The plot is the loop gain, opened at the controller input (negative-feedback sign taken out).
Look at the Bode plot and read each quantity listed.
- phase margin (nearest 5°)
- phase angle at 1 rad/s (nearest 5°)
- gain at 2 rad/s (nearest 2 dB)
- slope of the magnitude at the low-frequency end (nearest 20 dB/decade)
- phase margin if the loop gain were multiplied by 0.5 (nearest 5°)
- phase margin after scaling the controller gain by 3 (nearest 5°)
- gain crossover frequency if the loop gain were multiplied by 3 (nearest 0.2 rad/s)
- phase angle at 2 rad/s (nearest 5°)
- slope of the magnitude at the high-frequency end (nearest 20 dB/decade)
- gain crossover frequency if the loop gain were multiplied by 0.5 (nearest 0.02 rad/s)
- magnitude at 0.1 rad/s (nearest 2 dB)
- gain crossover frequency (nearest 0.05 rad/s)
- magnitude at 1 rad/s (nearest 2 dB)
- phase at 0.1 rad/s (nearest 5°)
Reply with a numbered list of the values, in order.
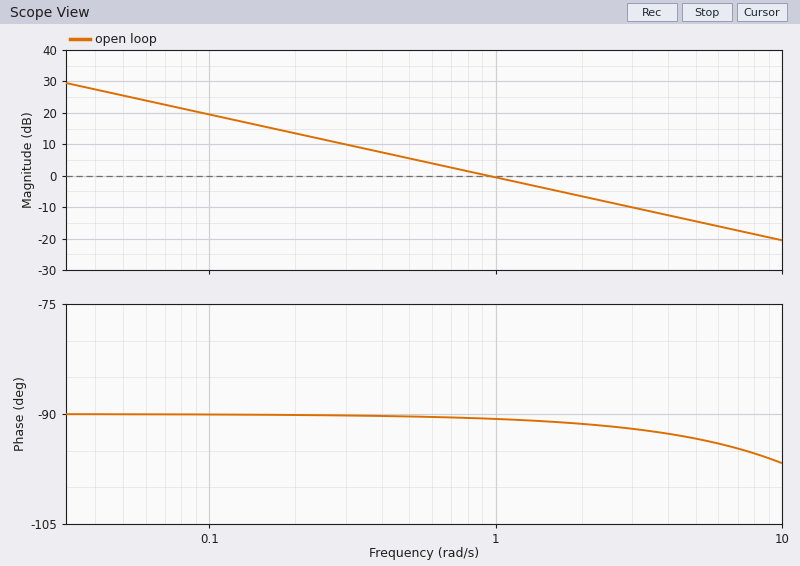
1. 90°
2. -90°
3. -6 dB
4. -20 dB/decade
5. 90°
6. 90°
7. 2.8 rad/s
8. -90°
9. -20 dB/decade
10. 0.48 rad/s
11. 20 dB
12. 0.95 rad/s
13. 0 dB
14. -90°
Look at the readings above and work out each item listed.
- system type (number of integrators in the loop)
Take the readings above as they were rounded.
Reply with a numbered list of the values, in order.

1. 1
